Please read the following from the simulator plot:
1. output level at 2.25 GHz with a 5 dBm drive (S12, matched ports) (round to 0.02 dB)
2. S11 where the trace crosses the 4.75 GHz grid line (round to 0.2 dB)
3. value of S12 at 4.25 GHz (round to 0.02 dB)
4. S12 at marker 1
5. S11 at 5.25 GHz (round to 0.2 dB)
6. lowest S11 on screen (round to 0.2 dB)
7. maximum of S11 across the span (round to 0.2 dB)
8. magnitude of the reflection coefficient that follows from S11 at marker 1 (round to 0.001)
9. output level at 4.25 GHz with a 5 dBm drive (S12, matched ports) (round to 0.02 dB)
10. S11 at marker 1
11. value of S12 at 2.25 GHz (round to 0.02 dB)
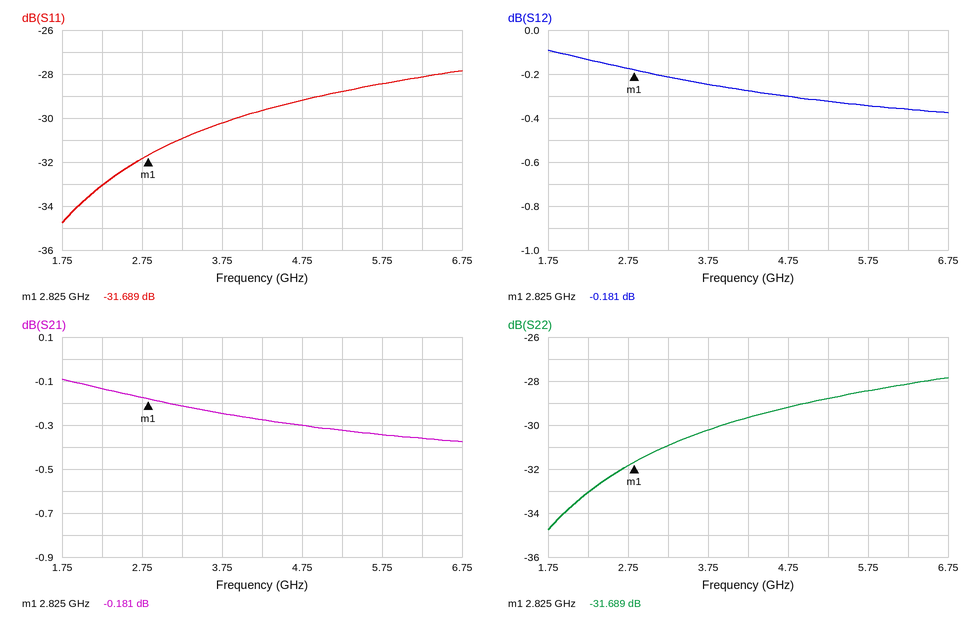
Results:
4.86 dBm
-29.2 dB
-0.28 dB
-0.181 dB
-28.8 dB
-34.8 dB
-27.8 dB
0.026
4.72 dBm
-31.689 dB
-0.14 dB
